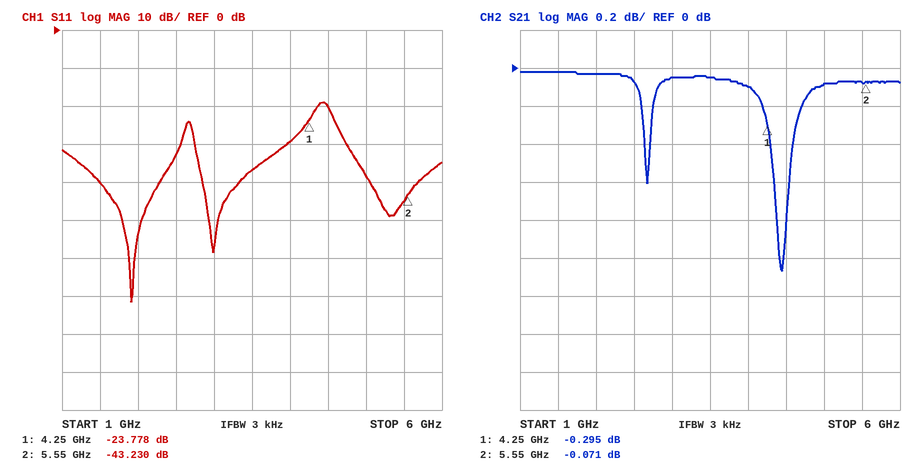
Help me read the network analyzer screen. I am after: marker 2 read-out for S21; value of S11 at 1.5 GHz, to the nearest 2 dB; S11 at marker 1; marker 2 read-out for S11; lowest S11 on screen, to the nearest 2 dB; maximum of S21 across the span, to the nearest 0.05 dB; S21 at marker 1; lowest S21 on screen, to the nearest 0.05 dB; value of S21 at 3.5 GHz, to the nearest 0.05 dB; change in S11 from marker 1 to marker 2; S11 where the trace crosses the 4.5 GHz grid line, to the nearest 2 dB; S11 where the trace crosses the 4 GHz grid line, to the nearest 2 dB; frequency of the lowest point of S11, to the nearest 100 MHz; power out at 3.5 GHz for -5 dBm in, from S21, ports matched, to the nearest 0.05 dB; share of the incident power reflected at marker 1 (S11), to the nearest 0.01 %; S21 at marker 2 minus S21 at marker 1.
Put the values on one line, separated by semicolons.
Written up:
-0.071 dB; -40 dB; -23.778 dB; -43.230 dB; -72 dB; 0.00 dB; -0.295 dB; -1.05 dB; -0.05 dB; -19.452 dB; -20 dB; -30 dB; 1.9 GHz; -5.05 dBm; 0.42 %; 0.224 dB
